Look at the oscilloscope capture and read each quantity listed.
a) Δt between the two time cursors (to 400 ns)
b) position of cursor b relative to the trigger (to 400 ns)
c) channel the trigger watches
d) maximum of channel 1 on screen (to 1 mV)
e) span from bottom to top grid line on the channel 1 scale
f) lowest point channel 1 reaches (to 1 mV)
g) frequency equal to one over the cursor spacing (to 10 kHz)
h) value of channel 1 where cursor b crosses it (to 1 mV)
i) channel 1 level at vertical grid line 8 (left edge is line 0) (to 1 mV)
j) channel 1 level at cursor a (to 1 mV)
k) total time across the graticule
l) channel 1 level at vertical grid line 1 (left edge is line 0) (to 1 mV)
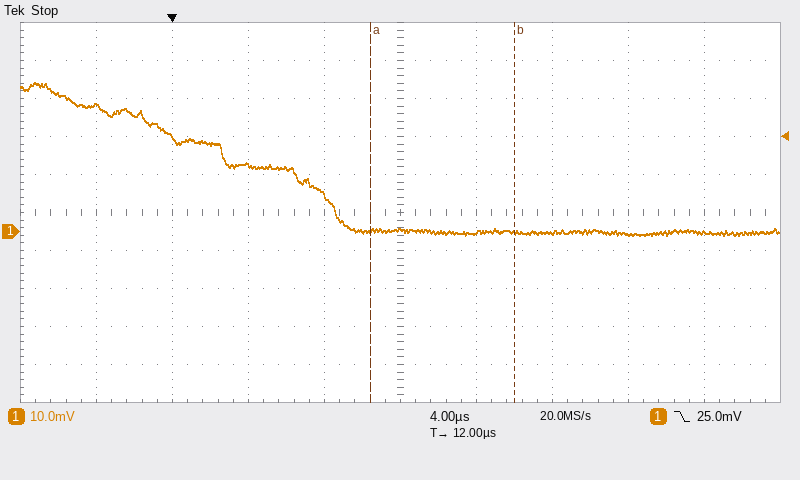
7.6 µs
+18.0 µs
channel 1
39 mV
100 mV
-1 mV
130 kHz
0 mV
-1 mV
0 mV
40 µs
33 mV
